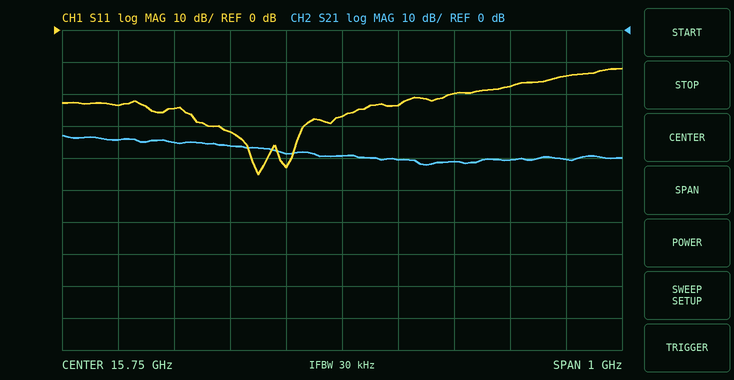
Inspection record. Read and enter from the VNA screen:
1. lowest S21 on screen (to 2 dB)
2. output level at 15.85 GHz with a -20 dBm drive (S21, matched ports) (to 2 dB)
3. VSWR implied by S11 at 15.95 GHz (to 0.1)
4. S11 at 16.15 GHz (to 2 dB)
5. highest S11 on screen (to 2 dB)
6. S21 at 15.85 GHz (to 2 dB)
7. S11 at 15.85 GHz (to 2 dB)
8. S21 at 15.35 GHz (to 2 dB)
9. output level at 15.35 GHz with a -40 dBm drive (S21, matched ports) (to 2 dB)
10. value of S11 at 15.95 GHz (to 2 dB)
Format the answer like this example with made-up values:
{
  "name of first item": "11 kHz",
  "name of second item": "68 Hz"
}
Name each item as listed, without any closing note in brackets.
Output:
{
  "lowest S21 on screen": "-42 dB",
  "output level at 15.85 GHz with a -20 dBm drive (S21, matched ports)": "-60 dBm",
  "VSWR implied by S11 at 15.95 GHz": "1.2",
  "S11 at 16.15 GHz": "-14 dB",
  "highest S11 on screen": "-12 dB",
  "S21 at 15.85 GHz": "-40 dB",
  "S11 at 15.85 GHz": "-24 dB",
  "S21 at 15.35 GHz": "-34 dB",
  "output level at 15.35 GHz with a -40 dBm drive (S21, matched ports)": "-74 dBm",
  "value of S11 at 15.95 GHz": "-20 dB"
}
